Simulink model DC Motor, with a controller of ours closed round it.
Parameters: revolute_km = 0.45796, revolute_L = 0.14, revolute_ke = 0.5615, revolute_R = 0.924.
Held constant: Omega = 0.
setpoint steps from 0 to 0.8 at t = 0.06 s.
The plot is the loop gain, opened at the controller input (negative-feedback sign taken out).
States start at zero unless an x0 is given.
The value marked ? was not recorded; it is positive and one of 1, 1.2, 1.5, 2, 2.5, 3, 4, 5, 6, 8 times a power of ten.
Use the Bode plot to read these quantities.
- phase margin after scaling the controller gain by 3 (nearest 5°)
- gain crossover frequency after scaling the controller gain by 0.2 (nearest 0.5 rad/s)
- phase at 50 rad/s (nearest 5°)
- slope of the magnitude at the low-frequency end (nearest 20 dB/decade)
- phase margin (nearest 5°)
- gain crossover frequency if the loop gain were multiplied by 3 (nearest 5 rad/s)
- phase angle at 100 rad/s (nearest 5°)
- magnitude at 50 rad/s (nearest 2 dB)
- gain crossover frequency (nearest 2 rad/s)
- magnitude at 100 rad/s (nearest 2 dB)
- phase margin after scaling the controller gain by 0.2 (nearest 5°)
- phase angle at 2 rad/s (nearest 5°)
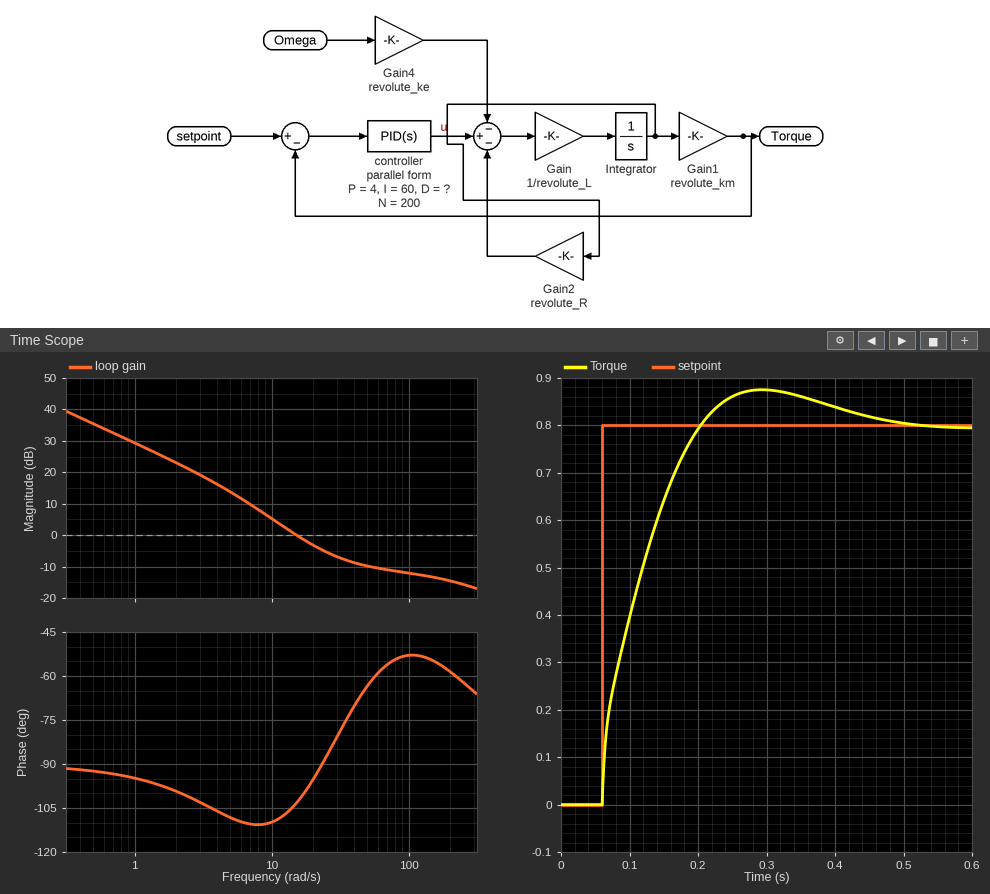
115°
5.0 rad/s
-65°
-20 dB/decade
75°
45 rad/s
-55°
-10 dB
16 rad/s
-12 dB
70°
-100°
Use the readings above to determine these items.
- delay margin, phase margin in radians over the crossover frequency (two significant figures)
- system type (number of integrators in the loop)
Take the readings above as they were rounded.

0.082 s
1
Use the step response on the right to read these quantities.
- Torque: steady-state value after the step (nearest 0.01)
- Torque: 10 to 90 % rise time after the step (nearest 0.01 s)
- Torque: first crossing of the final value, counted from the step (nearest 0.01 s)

0.80
0.11 s
0.14 s
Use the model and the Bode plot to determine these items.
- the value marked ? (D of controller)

0.06
